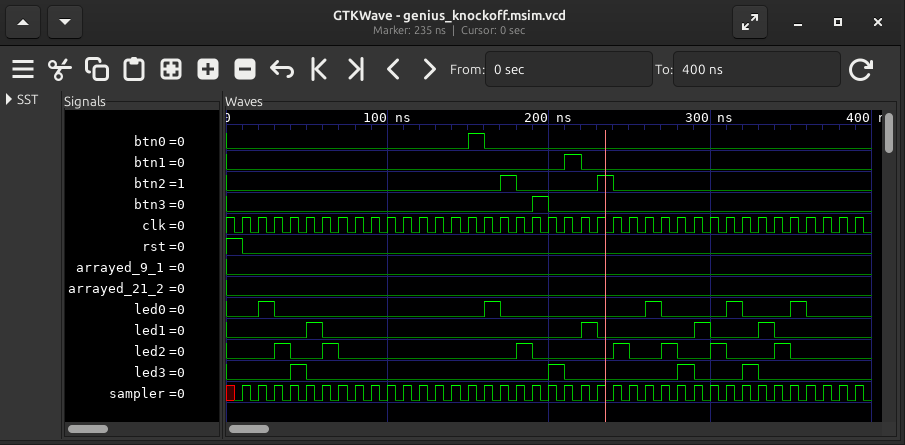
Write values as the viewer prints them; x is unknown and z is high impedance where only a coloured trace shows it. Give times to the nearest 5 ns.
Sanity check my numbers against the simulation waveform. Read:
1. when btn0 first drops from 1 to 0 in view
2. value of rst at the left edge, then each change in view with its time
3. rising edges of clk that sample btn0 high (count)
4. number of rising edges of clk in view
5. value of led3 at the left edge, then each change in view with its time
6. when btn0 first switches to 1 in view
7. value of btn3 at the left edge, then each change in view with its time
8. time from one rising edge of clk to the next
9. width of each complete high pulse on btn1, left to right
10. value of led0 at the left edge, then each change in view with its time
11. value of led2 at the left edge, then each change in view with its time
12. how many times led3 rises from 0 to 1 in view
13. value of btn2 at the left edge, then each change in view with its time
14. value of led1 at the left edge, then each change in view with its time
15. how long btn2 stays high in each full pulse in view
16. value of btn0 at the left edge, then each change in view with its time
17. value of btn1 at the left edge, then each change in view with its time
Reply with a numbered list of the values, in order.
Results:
1. 160 ns
2. 1, 0 at 10 ns
3. 1
4. 39
5. 0, 1 at 40 ns, 0 at 50 ns, 1 at 200 ns, 0 at 210 ns, 1 at 280 ns, 0 at 290 ns, 1 at 320 ns, 0 at 330 ns
6. 150 ns
7. 0, 1 at 190 ns, 0 at 200 ns
8. 10 ns
9. 10 ns
10. 0, 1 at 20 ns, 0 at 30 ns, 1 at 160 ns, 0 at 170 ns, 1 at 260 ns, 0 at 270 ns, 1 at 310 ns, 0 at 320 ns, 1 at 350 ns, 0 at 360 ns
11. 0, 1 at 30 ns, 0 at 40 ns, 1 at 60 ns, 0 at 70 ns, 1 at 180 ns, 0 at 190 ns, 1 at 240 ns, 0 at 250 ns, 1 at 270 ns, 0 at 280 ns, 1 at 300 ns, 0 at 310 ns, 1 at 340 ns, 0 at 350 ns
12. 4
13. 0, 1 at 170 ns, 0 at 180 ns, 1 at 230 ns, 0 at 240 ns
14. 0, 1 at 50 ns, 0 at 60 ns, 1 at 220 ns, 0 at 230 ns, 1 at 290 ns, 0 at 300 ns, 1 at 330 ns, 0 at 340 ns
15. 10 ns, 10 ns
16. 0, 1 at 150 ns, 0 at 160 ns
17. 0, 1 at 210 ns, 0 at 220 ns
